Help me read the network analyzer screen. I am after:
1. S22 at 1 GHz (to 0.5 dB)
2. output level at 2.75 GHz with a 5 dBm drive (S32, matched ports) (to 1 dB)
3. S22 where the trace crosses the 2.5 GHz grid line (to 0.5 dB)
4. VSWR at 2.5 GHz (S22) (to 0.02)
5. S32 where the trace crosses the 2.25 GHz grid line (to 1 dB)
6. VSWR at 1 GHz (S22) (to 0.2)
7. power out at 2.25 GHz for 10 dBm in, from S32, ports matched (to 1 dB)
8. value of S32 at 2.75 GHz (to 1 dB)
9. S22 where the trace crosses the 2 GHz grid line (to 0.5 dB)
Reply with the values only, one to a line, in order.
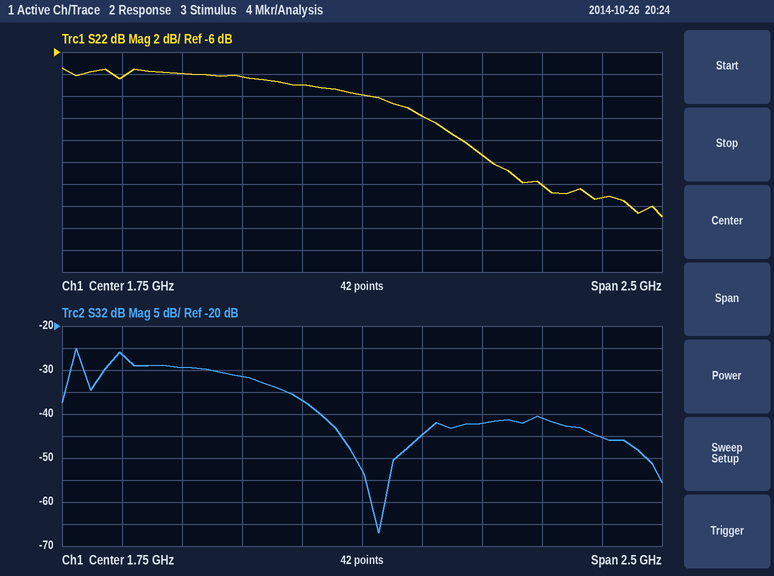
-8.0 dB
-40 dBm
-18.0 dB
1.28
-42 dB
2.4
-32 dBm
-45 dB
-12.0 dB
